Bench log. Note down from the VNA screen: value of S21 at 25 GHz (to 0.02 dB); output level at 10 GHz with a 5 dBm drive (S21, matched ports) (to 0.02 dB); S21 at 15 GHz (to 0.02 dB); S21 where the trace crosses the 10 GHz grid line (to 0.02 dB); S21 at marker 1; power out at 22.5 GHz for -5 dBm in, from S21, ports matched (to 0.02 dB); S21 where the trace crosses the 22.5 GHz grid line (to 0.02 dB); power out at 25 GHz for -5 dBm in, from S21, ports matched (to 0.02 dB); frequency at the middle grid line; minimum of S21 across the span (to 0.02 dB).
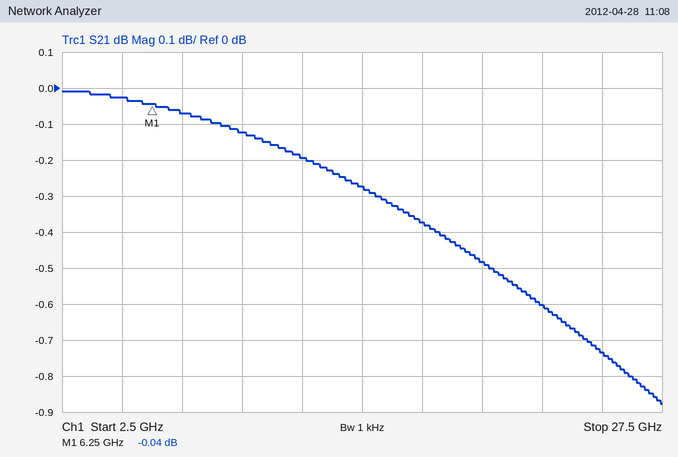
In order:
-0.74 dB
4.88 dBm
-0.28 dB
-0.12 dB
-0.04 dB
-5.60 dBm
-0.60 dB
-5.74 dBm
15 GHz
-0.88 dB
